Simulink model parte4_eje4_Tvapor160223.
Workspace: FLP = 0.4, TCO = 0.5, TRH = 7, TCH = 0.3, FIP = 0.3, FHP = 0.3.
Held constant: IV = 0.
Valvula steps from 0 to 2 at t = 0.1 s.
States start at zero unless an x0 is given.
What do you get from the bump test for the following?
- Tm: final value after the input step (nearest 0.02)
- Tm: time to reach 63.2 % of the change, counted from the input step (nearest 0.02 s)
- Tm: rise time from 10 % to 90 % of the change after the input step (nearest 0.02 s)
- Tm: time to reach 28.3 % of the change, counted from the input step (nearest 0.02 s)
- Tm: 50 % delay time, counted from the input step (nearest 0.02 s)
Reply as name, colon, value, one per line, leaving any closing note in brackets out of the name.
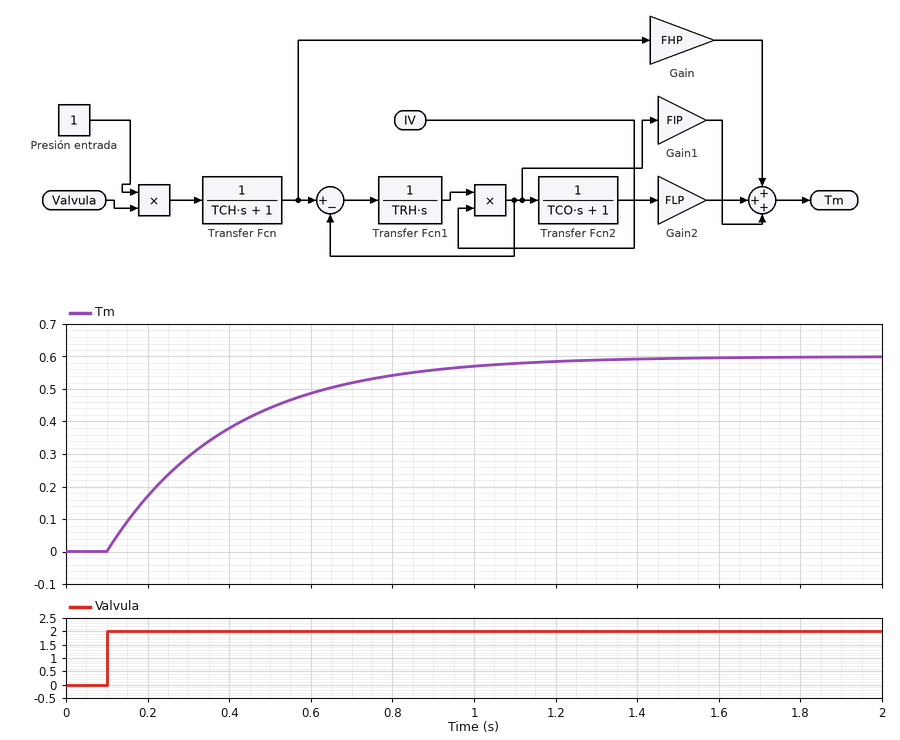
Tm: final value after the input step: 0.60
Tm: time to reach 63.2 % of the change, counted from the input step: 0.30 s
Tm: rise time from 10 % to 90 % of the change after the input step: 0.66 s
Tm: time to reach 28.3 % of the change, counted from the input step: 0.10 s
Tm: 50 % delay time, counted from the input step: 0.20 s
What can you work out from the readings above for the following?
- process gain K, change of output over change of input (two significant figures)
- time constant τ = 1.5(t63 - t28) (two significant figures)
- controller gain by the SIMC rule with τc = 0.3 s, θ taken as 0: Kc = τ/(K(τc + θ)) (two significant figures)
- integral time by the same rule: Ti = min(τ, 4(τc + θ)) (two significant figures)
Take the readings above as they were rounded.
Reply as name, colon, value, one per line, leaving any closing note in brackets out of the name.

process gain K, change of output over change of input: 0.30
time constant τ = 1.5(t63 - t28): 0.30 s
controller gain by the SIMC rule with τc = 0.3 s, θ taken as 0: Kc = τ/(K(τc + θ)): 3.3
integral time by the same rule: Ti = min(τ, 4(τc + θ)): 0.30 s
